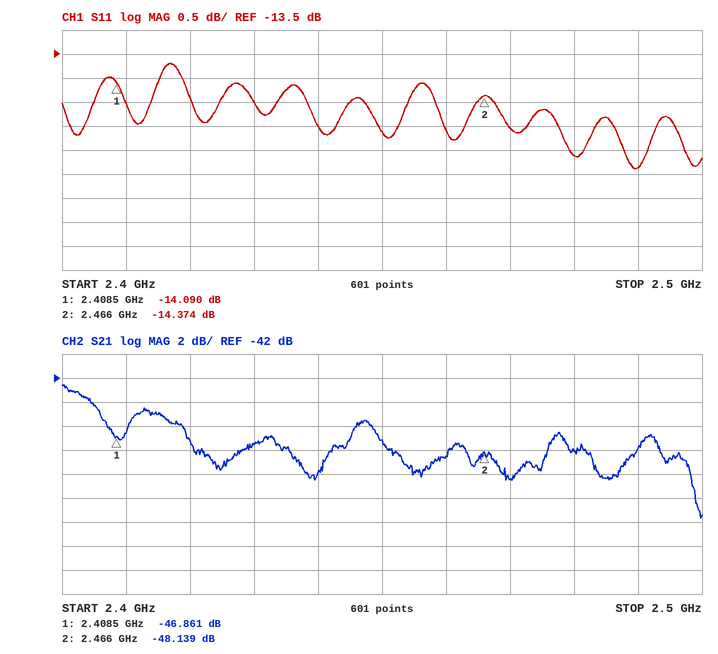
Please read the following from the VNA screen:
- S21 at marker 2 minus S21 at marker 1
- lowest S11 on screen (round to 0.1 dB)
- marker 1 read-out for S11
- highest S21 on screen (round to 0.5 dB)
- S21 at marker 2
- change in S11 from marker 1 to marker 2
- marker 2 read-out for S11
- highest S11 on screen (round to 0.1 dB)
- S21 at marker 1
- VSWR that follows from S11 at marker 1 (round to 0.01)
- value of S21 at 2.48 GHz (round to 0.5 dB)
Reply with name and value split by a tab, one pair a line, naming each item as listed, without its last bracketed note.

S21 at marker 2 minus S21 at marker 1	-1.278 dB
lowest S11 on screen	-15.9 dB
marker 1 read-out for S11	-14.090 dB
highest S21 on screen	-42.5 dB
S21 at marker 2	-48.139 dB
change in S11 from marker 1 to marker 2	-0.284 dB
marker 2 read-out for S11	-14.374 dB
highest S11 on screen	-13.7 dB
S21 at marker 1	-46.861 dB
VSWR that follows from S11 at marker 1	1.49
value of S21 at 2.48 GHz	-48.0 dB
